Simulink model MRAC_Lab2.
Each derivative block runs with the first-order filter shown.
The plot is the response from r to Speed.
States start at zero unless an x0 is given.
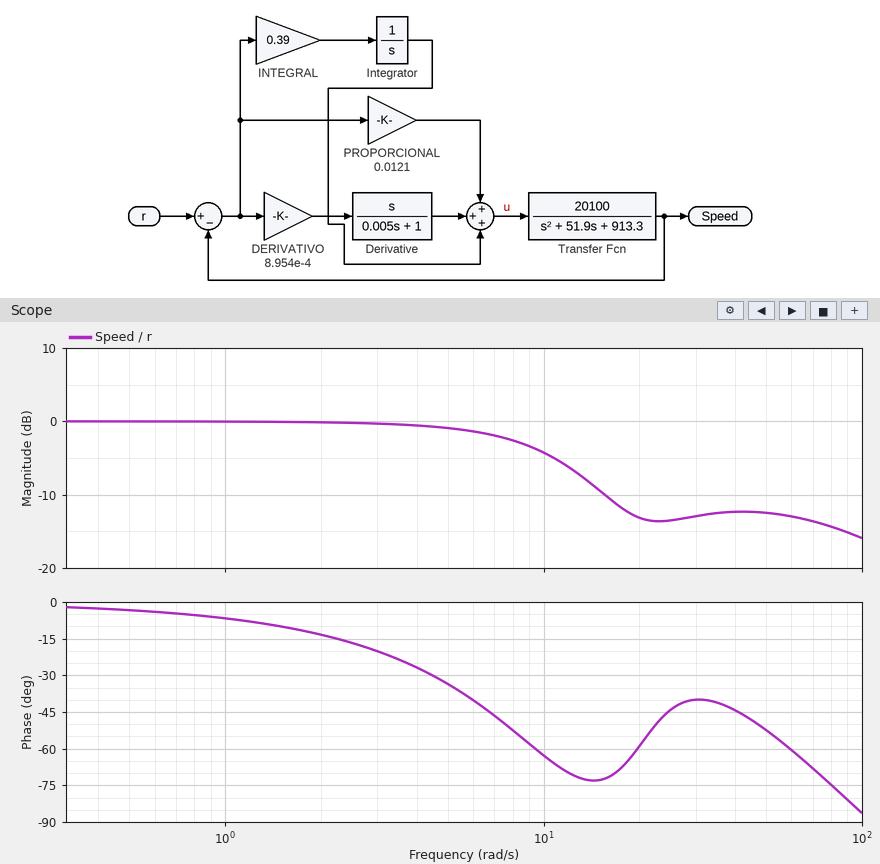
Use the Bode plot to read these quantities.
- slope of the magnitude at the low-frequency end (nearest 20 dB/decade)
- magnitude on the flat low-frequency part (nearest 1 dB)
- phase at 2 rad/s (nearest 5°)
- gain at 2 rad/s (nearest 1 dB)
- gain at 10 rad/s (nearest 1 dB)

0 dB/decade
0 dB
-15°
0 dB
-4 dB
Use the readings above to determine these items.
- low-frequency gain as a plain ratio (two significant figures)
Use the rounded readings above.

1.0
